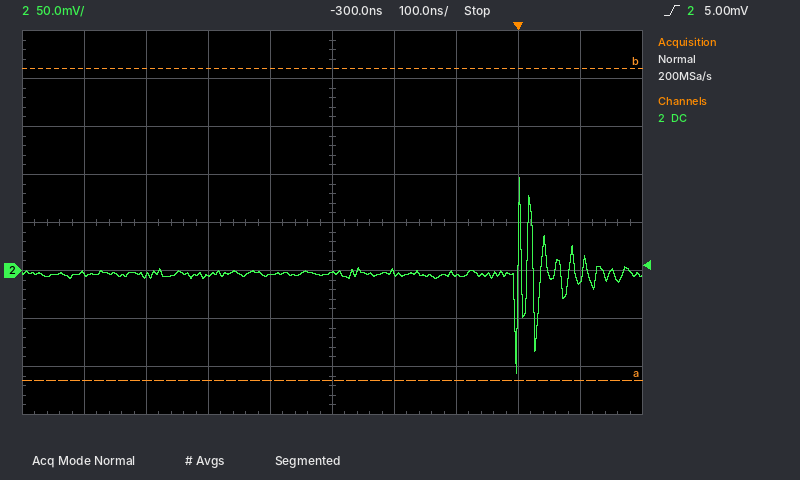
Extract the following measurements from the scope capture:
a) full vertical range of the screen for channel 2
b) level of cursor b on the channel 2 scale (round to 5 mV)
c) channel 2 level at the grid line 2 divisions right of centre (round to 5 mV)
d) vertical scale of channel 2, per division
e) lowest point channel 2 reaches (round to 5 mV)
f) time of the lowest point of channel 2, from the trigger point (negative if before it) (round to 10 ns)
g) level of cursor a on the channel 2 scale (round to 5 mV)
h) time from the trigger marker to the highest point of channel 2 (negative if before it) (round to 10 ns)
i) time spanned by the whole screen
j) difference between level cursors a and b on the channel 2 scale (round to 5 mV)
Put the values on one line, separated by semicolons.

400 mV; 210 mV; -5 mV; 50 mV; -105 mV; 0 ns; -115 mV; 0 ns; 1 µs; 325 mV
